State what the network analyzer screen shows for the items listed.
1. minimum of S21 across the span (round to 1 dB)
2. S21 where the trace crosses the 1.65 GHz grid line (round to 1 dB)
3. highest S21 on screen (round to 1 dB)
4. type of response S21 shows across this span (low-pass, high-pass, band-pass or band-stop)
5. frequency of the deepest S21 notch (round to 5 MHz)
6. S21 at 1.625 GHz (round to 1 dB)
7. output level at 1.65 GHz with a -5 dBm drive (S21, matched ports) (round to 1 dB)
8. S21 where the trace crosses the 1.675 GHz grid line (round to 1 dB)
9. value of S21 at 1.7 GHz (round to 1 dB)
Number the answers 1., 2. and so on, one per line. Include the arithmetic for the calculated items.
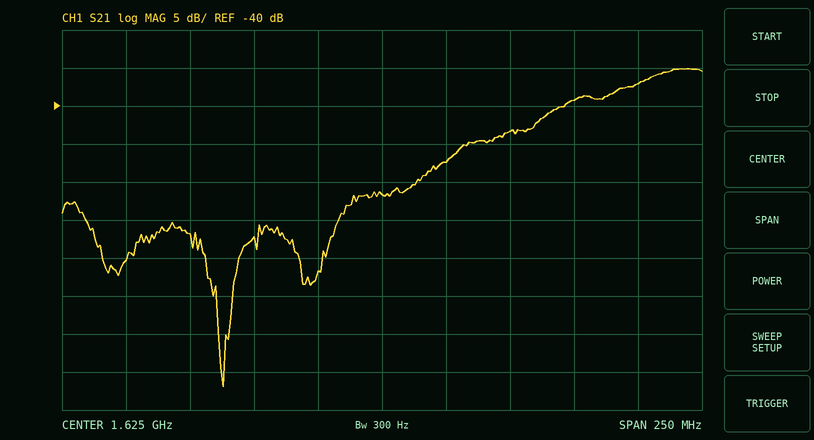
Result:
1. -77 dB
2. -47 dB
3. -35 dB
4. high-pass
5. 1.565 GHz
6. -52 dB
7. -5 dBm + (-47 dB) = -52 dBm
8. -43 dB
9. -39 dB
